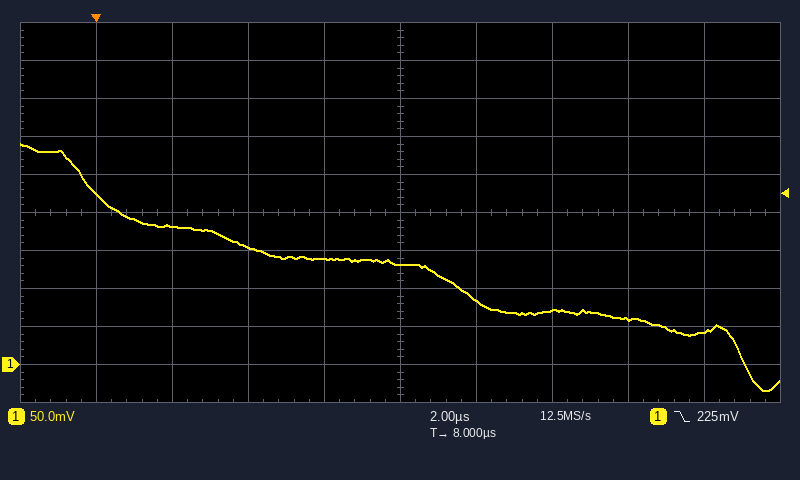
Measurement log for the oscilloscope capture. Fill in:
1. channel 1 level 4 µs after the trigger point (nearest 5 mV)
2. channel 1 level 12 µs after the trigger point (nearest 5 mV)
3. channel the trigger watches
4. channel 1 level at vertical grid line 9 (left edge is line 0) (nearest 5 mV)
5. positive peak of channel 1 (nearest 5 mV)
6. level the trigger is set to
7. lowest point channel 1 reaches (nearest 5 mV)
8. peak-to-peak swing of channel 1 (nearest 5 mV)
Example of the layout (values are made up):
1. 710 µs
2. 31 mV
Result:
1. 155 mV
2. 70 mV
3. channel 1
4. 45 mV
5. 290 mV
6. 225 mV
7. -35 mV
8. 325 mV
